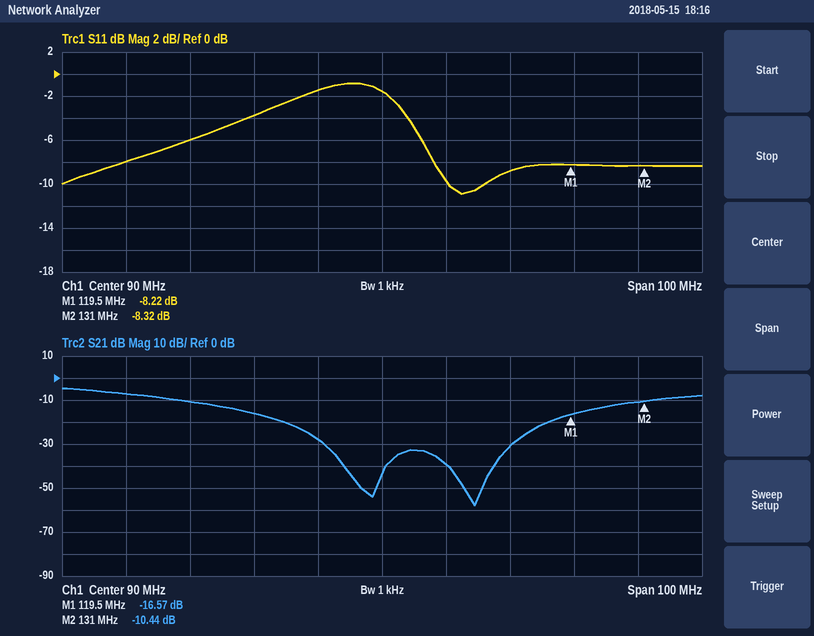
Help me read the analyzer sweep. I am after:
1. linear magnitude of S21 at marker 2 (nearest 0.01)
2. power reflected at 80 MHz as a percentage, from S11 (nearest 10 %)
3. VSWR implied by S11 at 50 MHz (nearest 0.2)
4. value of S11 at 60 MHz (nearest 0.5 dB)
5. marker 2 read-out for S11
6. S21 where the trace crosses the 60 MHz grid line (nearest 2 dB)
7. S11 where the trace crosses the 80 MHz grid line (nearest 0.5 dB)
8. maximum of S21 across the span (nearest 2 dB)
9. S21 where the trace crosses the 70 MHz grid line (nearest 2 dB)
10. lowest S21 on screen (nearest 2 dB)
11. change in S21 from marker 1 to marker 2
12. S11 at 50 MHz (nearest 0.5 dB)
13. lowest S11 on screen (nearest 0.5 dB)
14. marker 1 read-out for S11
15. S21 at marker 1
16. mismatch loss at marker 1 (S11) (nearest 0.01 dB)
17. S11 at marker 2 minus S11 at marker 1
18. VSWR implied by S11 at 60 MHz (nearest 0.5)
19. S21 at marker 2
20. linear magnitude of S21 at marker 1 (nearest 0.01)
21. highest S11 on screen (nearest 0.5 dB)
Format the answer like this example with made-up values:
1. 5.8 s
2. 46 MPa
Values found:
1. 0.30
2. 70 %
3. 2.4
4. -6.0 dB
5. -8.32 dB
6. -10 dB
7. -1.5 dB
8. -4 dB
9. -16 dB
10. -58 dB
11. 6.13 dB
12. -8.0 dB
13. -11.0 dB
14. -8.22 dB
15. -16.57 dB
16. 0.71 dB
17. -0.10 dB
18. 3.0
19. -10.44 dB
20. 0.15
21. -1.0 dB
